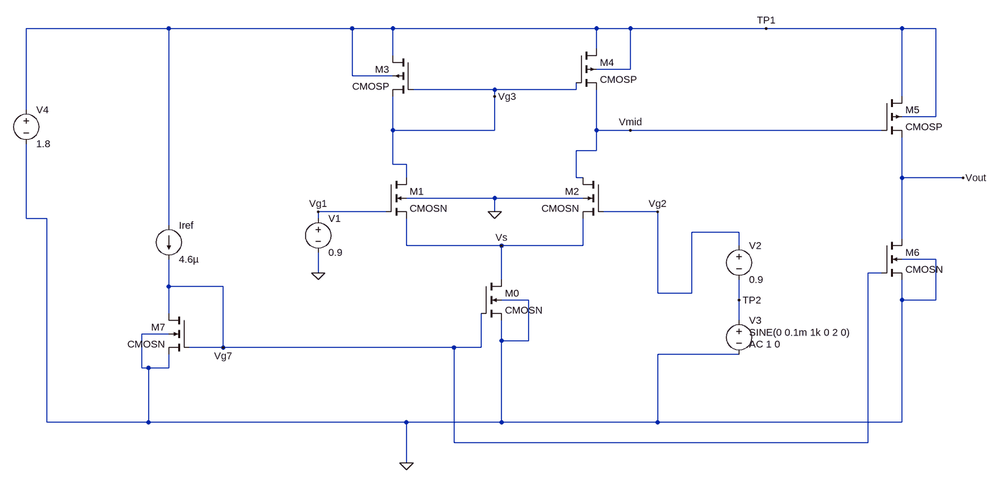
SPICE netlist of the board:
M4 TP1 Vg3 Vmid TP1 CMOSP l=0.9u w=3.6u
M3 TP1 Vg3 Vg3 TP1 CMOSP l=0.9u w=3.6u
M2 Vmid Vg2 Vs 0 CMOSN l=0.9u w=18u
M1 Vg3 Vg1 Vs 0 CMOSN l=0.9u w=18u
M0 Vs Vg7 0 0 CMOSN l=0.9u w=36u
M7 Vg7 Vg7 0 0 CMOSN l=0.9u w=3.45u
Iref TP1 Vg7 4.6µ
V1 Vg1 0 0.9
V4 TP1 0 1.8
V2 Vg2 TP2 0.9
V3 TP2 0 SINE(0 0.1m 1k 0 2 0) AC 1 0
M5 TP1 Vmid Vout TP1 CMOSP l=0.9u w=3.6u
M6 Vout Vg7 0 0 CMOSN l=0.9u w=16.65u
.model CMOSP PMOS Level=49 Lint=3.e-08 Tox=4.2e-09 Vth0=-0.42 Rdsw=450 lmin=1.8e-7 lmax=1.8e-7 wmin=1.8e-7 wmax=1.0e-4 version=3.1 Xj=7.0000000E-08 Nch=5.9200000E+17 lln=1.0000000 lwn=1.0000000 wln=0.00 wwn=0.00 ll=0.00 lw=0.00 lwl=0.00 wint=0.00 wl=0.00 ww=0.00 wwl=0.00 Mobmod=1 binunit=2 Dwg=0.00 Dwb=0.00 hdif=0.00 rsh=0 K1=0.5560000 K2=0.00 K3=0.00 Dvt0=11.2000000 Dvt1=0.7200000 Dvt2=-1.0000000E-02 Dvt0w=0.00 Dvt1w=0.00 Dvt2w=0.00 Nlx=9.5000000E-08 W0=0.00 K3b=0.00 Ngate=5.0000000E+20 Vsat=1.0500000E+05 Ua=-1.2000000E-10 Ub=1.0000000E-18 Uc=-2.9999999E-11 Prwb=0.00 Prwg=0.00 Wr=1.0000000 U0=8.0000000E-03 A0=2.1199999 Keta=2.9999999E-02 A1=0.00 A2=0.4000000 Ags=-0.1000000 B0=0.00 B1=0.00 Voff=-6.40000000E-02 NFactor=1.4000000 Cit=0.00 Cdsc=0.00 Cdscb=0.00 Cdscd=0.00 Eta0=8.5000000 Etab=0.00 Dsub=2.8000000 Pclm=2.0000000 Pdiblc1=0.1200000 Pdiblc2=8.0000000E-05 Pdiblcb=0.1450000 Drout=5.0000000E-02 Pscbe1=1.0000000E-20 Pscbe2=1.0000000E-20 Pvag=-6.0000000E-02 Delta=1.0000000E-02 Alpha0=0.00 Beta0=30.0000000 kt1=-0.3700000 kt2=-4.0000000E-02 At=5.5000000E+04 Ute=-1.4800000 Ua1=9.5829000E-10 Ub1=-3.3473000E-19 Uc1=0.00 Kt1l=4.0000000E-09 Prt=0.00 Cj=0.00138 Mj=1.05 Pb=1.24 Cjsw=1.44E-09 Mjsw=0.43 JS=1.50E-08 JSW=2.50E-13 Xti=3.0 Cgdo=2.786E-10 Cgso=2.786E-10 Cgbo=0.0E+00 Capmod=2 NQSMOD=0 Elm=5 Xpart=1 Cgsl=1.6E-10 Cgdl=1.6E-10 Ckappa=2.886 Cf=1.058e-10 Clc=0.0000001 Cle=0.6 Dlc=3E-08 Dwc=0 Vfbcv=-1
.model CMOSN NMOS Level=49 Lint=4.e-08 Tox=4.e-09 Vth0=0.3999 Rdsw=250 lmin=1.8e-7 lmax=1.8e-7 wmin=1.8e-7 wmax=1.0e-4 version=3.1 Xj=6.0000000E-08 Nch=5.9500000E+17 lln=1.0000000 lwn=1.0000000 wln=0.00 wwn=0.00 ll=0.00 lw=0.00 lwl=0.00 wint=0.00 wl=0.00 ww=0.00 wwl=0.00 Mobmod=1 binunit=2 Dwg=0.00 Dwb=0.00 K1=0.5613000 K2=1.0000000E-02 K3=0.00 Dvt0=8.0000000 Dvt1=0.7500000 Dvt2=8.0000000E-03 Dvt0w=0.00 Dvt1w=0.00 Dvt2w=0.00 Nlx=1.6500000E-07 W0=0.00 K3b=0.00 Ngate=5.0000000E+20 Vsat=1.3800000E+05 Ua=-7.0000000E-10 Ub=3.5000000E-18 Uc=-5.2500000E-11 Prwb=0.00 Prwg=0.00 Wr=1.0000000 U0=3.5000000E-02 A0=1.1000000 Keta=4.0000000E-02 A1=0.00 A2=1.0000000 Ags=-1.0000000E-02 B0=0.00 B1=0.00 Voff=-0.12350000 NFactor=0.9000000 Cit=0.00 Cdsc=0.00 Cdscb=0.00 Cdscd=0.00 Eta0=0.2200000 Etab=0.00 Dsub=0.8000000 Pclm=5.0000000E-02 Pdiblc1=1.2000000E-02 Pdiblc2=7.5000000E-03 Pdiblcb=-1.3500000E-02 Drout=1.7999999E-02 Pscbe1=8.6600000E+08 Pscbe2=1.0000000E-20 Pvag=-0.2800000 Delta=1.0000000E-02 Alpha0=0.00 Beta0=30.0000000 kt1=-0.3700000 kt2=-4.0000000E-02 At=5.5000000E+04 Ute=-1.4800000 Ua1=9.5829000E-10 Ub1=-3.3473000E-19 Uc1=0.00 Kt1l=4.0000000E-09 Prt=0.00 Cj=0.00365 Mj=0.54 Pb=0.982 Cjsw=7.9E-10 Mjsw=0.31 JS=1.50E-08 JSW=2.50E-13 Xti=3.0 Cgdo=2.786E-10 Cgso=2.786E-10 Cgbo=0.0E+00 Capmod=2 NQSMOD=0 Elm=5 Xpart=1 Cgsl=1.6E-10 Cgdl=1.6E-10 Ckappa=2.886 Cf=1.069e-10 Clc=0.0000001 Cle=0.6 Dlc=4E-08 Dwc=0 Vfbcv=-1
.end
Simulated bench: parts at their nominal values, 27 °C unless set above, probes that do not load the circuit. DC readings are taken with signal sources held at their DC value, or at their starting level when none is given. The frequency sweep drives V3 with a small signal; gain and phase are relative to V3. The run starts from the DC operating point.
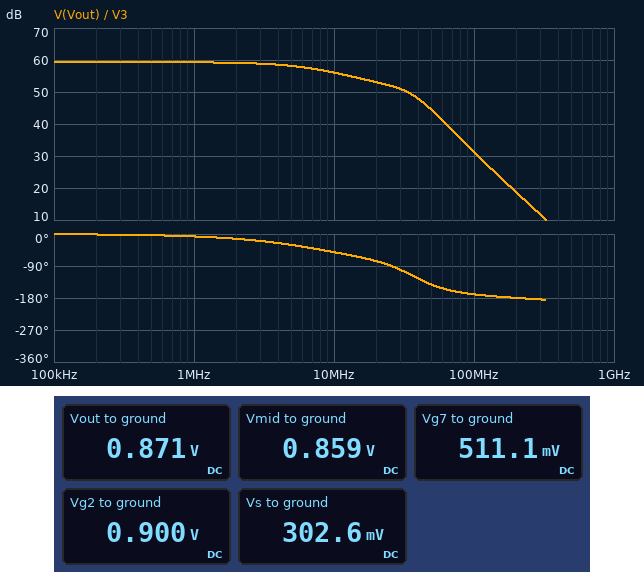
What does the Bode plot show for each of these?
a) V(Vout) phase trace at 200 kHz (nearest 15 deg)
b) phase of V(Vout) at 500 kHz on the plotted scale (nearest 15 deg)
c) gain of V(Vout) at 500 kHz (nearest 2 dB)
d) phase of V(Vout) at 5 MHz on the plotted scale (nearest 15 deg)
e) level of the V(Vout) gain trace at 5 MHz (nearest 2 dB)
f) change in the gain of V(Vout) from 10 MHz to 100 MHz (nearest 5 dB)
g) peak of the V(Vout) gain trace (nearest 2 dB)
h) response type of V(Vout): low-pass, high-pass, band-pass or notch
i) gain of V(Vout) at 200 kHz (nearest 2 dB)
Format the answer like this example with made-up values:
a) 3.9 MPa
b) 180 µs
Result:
a) 0 deg
b) 0 deg
c) 60 dB
d) -30 deg
e) 58 dB
f) -25 dB
g) 60 dB
h) low-pass
i) 60 dB
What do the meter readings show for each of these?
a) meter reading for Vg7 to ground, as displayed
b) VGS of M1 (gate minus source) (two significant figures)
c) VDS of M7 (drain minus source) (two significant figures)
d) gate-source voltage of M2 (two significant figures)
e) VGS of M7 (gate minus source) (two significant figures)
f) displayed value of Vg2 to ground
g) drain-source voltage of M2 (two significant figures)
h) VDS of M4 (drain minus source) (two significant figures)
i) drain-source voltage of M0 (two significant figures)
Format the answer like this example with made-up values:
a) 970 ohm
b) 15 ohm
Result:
a) 511.1 mV
b) 600 mV
c) 510 mV
d) 600 mV
e) 510 mV
f) 0.900 V
g) 560 mV
h) 940 mV
i) 300 mV
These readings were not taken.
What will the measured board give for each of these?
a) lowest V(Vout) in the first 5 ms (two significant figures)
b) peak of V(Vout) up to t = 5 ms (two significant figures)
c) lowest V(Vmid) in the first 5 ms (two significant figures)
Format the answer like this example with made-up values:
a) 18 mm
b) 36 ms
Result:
a) 780 mV
b) 960 mV
c) 850 mV
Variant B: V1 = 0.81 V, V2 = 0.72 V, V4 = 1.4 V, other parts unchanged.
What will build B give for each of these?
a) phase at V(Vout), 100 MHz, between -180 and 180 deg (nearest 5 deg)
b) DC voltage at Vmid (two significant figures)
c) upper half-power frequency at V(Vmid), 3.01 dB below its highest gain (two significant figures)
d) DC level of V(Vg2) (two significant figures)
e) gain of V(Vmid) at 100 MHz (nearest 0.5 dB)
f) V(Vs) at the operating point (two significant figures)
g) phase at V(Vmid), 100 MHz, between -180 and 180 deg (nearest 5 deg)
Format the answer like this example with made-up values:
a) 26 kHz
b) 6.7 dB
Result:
a) -145 deg
b) 1.3 V
c) 300 MHz
d) 720 mV
e) 0.5 dB
f) 200 mV
g) 160 deg
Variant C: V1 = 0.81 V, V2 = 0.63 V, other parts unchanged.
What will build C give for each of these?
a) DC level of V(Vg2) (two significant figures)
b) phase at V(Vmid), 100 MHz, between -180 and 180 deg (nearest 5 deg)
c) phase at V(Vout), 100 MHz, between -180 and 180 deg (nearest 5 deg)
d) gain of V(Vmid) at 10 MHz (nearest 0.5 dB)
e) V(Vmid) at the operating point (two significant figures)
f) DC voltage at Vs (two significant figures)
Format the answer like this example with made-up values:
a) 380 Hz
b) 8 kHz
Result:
a) 630 mV
b) 155 deg
c) -150 deg
d) -12.0 dB
e) 1.8 V
f) 200 mV
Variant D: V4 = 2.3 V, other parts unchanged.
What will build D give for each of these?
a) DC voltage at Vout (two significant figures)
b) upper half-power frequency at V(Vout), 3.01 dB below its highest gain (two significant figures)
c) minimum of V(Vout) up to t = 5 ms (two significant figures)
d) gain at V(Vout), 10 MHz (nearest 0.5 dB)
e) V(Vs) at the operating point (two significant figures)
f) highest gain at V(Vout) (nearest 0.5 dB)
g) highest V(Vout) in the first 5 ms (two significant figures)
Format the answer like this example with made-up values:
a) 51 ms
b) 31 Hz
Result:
a) 1.1 V
b) 9.2 MHz
c) 1.0 V
d) 56.5 dB
e) 310 mV
f) 60.0 dB
g) 1.2 V
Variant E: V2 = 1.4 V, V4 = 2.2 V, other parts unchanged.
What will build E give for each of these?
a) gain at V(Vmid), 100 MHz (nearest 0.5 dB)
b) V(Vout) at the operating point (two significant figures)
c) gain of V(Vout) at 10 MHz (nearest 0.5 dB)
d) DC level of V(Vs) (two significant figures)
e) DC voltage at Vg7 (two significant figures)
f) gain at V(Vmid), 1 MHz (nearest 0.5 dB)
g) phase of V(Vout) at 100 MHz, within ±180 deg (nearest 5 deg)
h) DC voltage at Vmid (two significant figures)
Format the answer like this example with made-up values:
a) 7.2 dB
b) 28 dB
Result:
a) -18.5 dB
b) 2.1 V
c) -59.0 dB
d) 310 mV
e) 510 mV
f) -37.5 dB
g) -105 deg
h) 320 mV
